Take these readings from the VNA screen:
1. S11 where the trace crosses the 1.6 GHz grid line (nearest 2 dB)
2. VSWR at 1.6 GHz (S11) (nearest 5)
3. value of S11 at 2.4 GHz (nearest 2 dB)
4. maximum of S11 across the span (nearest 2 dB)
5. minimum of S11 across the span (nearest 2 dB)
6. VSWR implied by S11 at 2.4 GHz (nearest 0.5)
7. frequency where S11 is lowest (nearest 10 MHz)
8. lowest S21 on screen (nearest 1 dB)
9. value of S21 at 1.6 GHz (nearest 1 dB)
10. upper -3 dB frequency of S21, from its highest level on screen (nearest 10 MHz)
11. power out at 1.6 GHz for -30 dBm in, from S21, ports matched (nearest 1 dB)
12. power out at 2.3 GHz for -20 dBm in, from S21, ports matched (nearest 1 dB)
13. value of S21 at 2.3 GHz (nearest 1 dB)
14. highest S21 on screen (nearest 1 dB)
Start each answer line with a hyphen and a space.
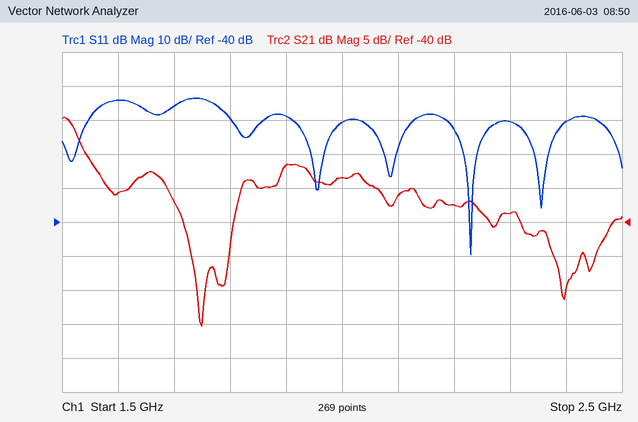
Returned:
- -4 dB
- 5
- -10 dB
- -4 dB
- -50 dB
- 2.0
- 2.23 GHz
- -55 dB
- -36 dB
- 1.53 GHz
- -66 dBm
- -59 dBm
- -39 dB
- -25 dB
